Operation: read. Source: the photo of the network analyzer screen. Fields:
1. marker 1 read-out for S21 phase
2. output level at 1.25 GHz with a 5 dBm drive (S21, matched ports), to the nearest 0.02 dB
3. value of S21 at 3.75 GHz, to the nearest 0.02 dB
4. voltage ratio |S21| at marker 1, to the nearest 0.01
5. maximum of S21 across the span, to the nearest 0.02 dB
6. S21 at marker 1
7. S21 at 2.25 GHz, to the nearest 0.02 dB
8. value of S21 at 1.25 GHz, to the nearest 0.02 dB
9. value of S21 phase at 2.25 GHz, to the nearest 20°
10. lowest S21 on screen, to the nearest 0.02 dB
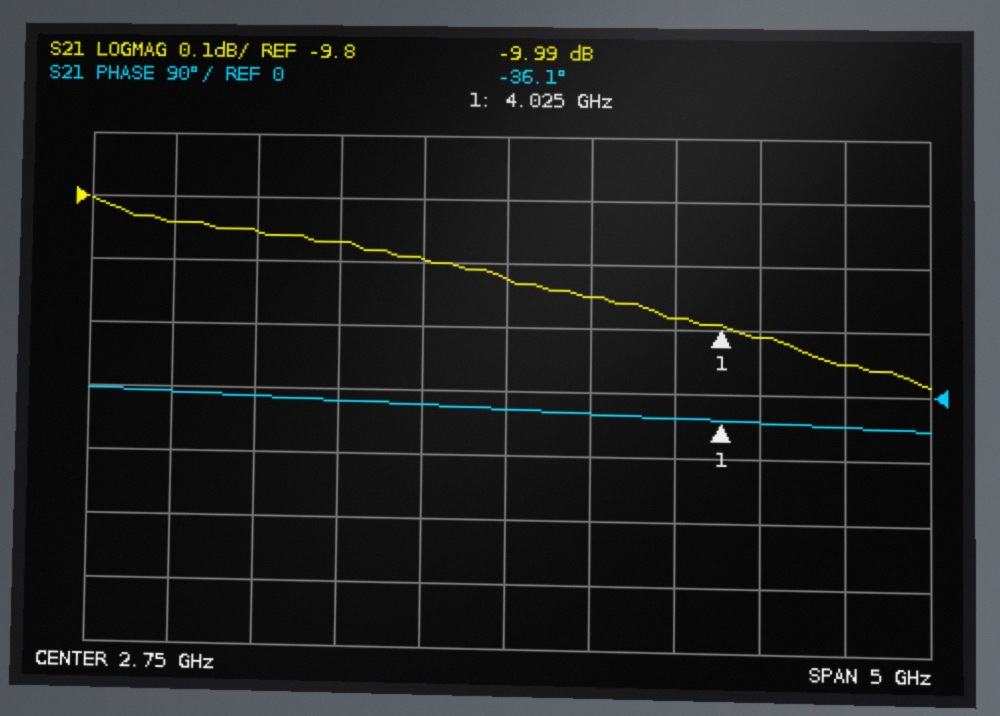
-36.1°
-4.86 dBm
-9.98 dB
0.32
-9.80 dB
-9.99 dB
-9.90 dB
-9.86 dB
-20°
-10.08 dB
